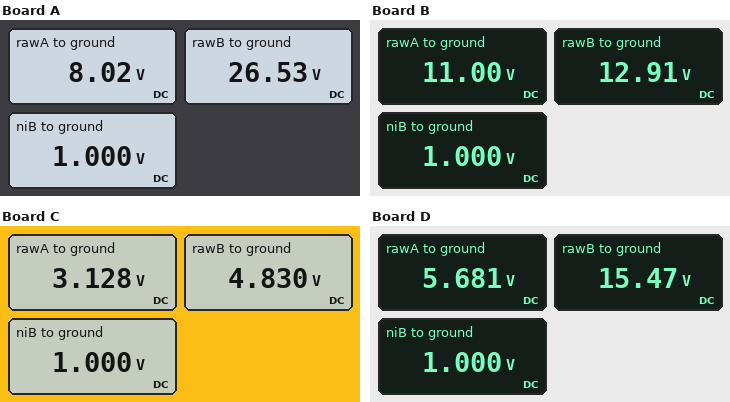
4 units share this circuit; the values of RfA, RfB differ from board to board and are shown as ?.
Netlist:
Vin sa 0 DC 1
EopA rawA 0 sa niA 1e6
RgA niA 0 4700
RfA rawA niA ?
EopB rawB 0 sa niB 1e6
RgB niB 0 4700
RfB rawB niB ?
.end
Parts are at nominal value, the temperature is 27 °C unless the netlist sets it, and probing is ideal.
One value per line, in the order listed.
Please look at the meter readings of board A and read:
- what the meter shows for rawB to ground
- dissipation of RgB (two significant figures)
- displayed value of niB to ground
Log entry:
26.53 V
210 µW
1.000 V
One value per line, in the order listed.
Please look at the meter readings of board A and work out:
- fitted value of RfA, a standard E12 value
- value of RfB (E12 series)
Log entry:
33 kΩ
120 kΩ
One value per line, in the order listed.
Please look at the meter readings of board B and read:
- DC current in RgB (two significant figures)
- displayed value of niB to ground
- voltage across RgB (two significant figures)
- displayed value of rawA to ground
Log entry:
210 µA
1.000 V
1.0 V
11.00 V
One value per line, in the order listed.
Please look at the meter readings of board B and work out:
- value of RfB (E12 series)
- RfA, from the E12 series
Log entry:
56 kΩ
47 kΩ
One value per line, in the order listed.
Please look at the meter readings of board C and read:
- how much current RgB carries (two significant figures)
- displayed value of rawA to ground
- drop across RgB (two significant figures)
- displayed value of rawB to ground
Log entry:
210 µA
3.128 V
1.0 V
4.830 V
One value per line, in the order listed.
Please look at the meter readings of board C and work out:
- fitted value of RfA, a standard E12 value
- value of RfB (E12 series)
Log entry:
10 kΩ
18 kΩ
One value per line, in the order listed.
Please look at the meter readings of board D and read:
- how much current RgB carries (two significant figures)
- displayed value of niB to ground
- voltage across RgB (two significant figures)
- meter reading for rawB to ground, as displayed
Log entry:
210 µA
1.000 V
1.0 V
15.47 V
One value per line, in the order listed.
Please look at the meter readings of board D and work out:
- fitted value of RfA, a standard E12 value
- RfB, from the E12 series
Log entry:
22 kΩ
68 kΩ
